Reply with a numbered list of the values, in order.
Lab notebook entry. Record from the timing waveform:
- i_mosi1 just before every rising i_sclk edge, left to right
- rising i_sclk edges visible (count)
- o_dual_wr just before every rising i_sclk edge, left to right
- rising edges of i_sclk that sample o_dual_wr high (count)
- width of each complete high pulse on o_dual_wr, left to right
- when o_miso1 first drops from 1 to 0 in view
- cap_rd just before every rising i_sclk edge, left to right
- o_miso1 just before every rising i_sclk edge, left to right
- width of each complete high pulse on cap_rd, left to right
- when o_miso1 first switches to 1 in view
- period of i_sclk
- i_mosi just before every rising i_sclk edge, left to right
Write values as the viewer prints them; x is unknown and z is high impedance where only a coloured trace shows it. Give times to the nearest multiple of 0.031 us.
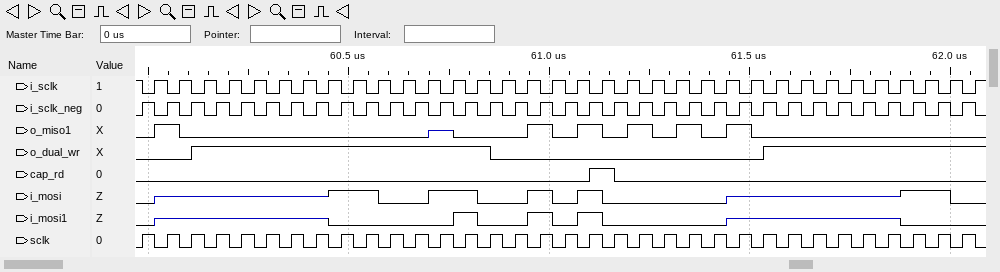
1. 0 z z z z z z z 0 0 0 0 0 1 0 0 1 0 1 0 0 0 0 0 z z z z z z z 0 0 0
2. 34
3. 0 0 1 1 1 1 1 1 1 1 1 1 1 1 0 0 0 0 0 0 0 0 0 0 0 1 1 1 1 1 1 1 1 1
4. 21
5. 0.744 us
6. 60.078 us
7. 0 0 0 0 0 0 0 0 0 0 0 0 0 0 0 0 0 0 1 0 0 0 0 0 0 0 0 0 0 0 0 0 0 0
8. 0 1 0 0 0 0 0 0 0 0 0 0 z 0 0 0 1 0 1 0 1 0 1 0 1 0 0 0 0 0 0 0 0 0
9. 0.062 us
10. 60.016 us
11. 0.062 us
12. 0 z z z z z z z 1 1 0 0 1 1 0 0 1 0 1 0 0 0 0 0 z z z z z z z 1 1 0
